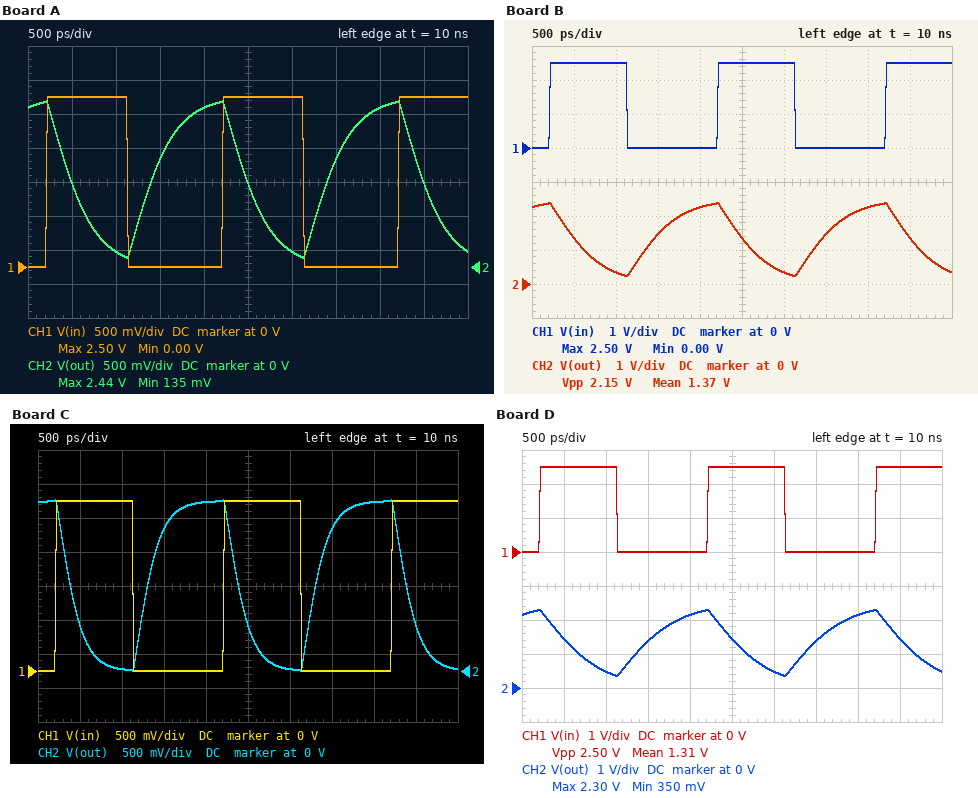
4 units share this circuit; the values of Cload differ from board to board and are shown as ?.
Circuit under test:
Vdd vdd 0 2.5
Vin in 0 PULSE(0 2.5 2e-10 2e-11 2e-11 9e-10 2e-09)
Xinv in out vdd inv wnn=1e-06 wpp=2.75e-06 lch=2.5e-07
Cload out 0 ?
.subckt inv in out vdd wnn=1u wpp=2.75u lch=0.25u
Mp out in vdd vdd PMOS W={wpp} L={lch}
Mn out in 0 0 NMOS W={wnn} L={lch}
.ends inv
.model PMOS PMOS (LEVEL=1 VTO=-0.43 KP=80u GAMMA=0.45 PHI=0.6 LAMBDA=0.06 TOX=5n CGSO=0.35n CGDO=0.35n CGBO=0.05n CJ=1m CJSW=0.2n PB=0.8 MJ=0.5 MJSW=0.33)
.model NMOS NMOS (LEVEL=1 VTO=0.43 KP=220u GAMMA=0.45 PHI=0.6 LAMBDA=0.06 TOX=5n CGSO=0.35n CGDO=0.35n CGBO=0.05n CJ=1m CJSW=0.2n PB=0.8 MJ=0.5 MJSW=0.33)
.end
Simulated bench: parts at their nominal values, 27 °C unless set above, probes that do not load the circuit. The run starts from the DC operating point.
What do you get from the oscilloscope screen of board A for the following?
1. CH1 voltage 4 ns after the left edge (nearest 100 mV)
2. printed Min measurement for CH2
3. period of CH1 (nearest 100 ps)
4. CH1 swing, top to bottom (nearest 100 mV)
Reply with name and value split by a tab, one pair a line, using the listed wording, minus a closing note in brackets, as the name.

CH1 voltage 4 ns after the left edge	0 V
printed Min measurement for CH2	135 mV
period of CH1	2.0 ns
CH1 swing, top to bottom	2.5 V
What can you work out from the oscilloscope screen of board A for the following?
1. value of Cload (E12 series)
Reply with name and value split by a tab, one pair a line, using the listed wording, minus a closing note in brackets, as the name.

value of Cload	470 fF
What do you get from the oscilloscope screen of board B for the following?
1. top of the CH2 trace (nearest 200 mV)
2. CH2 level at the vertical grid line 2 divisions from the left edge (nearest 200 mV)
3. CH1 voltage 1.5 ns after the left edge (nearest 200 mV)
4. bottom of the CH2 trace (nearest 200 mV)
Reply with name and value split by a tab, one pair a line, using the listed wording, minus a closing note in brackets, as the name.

top of the CH2 trace	2.4 V
CH2 level at the vertical grid line 2 divisions from the left edge	400 mV
CH1 voltage 1.5 ns after the left edge	0 V
bottom of the CH2 trace	200 mV
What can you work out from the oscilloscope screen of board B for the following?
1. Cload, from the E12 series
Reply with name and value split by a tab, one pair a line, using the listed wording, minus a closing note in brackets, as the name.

Cload, from the E12 series	560 fF
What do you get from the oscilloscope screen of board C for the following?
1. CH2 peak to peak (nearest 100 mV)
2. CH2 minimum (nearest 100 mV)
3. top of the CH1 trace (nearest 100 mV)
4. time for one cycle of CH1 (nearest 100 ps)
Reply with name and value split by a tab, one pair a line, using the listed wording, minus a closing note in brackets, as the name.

CH2 peak to peak	2.5 V
CH2 minimum	0 V
top of the CH1 trace	2.5 V
time for one cycle of CH1	2.0 ns
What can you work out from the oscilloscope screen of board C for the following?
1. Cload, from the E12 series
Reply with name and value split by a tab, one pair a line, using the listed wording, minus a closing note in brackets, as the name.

Cload, from the E12 series	270 fF
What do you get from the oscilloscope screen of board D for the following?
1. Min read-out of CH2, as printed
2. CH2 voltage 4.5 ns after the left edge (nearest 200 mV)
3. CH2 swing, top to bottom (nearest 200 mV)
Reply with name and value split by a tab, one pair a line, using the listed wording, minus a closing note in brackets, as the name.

Min read-out of CH2, as printed	350 mV
CH2 voltage 4.5 ns after the left edge	1.4 V
CH2 swing, top to bottom	2.0 V
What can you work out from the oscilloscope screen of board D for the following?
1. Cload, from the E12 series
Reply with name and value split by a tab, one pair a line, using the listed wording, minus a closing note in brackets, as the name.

Cload, from the E12 series	680 fF
